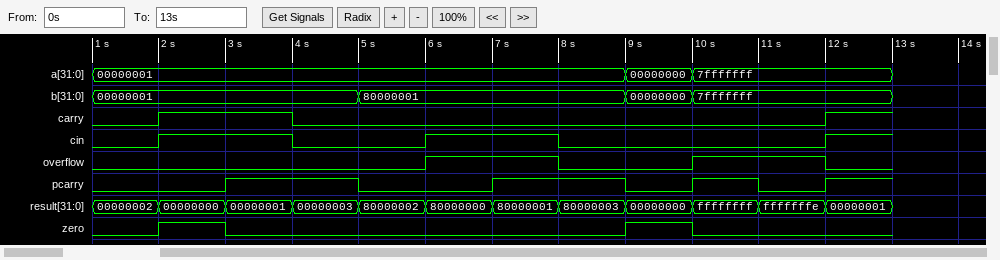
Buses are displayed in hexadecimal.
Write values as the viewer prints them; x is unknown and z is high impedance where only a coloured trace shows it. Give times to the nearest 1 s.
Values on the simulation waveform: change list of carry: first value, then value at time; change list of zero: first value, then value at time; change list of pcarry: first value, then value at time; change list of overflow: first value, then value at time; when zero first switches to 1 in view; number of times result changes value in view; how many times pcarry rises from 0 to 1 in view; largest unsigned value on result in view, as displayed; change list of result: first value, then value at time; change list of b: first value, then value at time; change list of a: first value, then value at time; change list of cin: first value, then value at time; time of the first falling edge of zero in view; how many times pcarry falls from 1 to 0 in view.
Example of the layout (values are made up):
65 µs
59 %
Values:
0, 1 at 2 s, 0 at 4 s, 1 at 12 s
0, 1 at 2 s, 0 at 3 s, 1 at 9 s, 0 at 10 s
0, 1 at 3 s, 0 at 5 s, 1 at 7 s, 0 at 9 s, 1 at 10 s, 0 at 11 s, 1 at 12 s
0, 1 at 6 s, 0 at 8 s, 1 at 10 s, 0 at 12 s
2 s
11
4
ffffffff
00000002, 00000000 at 2 s, 00000001 at 3 s, 00000003 at 4 s, 80000002 at 5 s, 80000000 at 6 s, 80000001 at 7 s, 80000003 at 8 s, 00000000 at 9 s, ffffffff at 10 s, fffffffe at 11 s, 00000001 at 12 s
00000001, 80000001 at 5 s, 00000000 at 9 s, 7fffffff at 10 s
00000001, 00000000 at 9 s, 7fffffff at 10 s
0, 1 at 2 s, 0 at 4 s, 1 at 6 s, 0 at 8 s, 1 at 12 s
3 s
3
